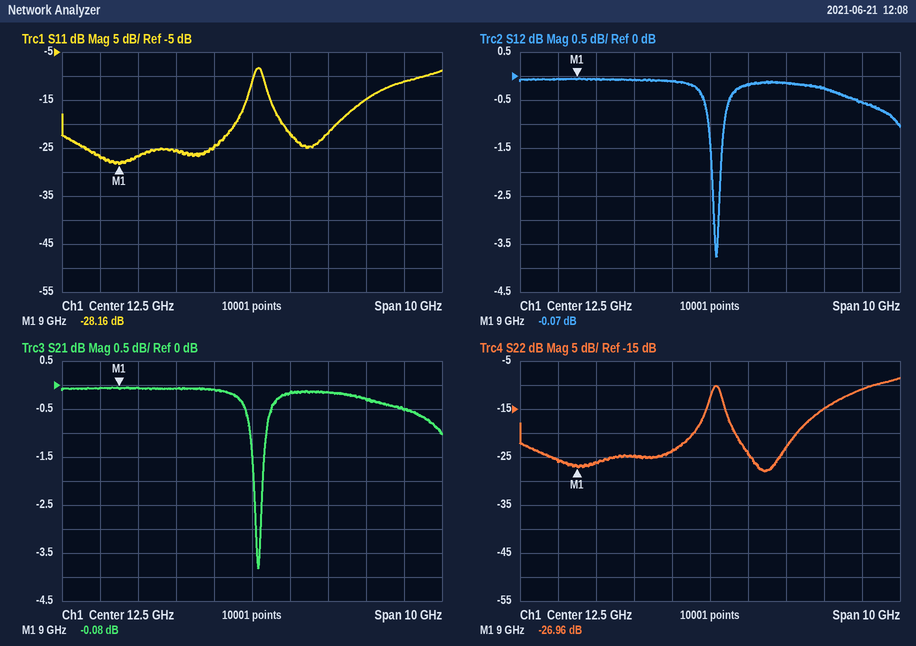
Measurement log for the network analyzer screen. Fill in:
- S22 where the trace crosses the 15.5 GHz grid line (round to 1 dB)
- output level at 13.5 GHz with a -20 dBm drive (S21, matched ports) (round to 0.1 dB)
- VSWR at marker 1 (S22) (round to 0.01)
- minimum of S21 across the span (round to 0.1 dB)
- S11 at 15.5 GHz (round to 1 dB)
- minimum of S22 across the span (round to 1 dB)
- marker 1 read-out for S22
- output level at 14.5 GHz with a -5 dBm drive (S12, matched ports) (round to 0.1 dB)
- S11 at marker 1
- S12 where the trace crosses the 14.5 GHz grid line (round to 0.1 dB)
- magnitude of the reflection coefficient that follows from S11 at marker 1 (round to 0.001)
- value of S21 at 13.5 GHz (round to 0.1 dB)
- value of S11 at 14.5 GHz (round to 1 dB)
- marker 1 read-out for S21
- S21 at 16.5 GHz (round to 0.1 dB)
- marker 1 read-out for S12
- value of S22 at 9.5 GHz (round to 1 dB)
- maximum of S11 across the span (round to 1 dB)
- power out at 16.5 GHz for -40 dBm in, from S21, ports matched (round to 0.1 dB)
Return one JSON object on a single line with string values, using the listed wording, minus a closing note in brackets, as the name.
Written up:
{"S22 where the trace crosses the 15.5 GHz grid line": "-15 dB", "output level at 13.5 GHz with a -20 dBm drive (S21, matched ports)": "-20.2 dBm", "VSWR at marker 1 (S22)": "1.09", "minimum of S21 across the span": "-3.8 dB", "S11 at 15.5 GHz": "-15 dB", "minimum of S22 across the span": "-28 dB", "marker 1 read-out for S22": "-26.96 dB", "output level at 14.5 GHz with a -5 dBm drive (S12, matched ports)": "-5.1 dBm", "S11 at marker 1": "-28.16 dB", "S12 where the trace crosses the 14.5 GHz grid line": "-0.1 dB", "magnitude of the reflection coefficient that follows from S11 at marker 1": "0.039", "value of S21 at 13.5 GHz": "-0.2 dB", "value of S11 at 14.5 GHz": "-22 dB", "marker 1 read-out for S21": "-0.08 dB", "S21 at 16.5 GHz": "-0.5 dB", "marker 1 read-out for S12": "-0.07 dB", "value of S22 at 9.5 GHz": "-26 dB", "maximum of S11 across the span": "-8 dB", "power out at 16.5 GHz for -40 dBm in, from S21, ports matched": "-40.5 dBm"}
